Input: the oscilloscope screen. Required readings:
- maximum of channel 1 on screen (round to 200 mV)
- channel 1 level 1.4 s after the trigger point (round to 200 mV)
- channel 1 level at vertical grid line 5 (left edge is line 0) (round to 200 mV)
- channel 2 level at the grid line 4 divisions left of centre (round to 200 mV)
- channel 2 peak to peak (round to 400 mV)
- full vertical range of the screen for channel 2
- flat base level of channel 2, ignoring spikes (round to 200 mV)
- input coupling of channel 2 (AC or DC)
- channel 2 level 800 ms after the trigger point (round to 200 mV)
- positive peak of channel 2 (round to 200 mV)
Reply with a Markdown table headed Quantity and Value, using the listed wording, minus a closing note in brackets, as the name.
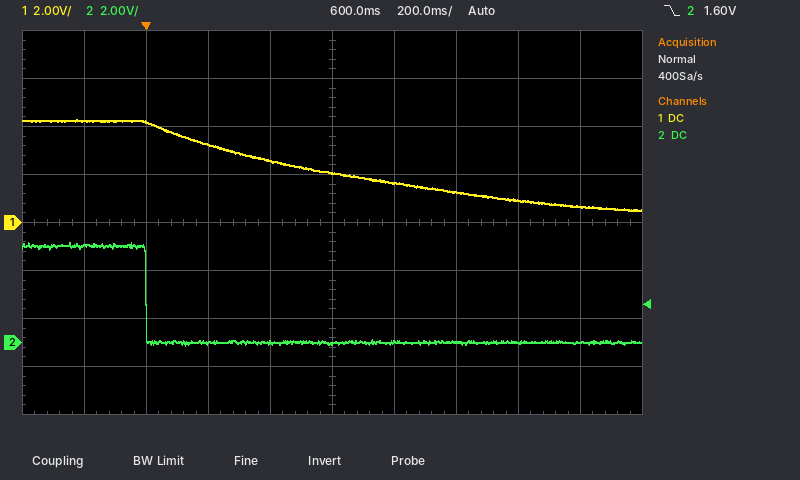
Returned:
| Quantity | Value |
|---|---|
| maximum of channel 1 on screen | 4.2 V |
| channel 1 level 1.4 s after the trigger point | 600 mV |
| channel 1 level at vertical grid line 5 (left edge is line 0) | 2.0 V |
| channel 2 level at the grid line 4 divisions left of centre | 4.0 V |
| channel 2 peak to peak | 4.4 V |
| full vertical range of the screen for channel 2 | 16 V |
| flat base level of channel 2, ignoring spikes | 0.0 V |
| input coupling of channel 2 | DC |
| channel 2 level 800 ms after the trigger point | 0.0 V |
| positive peak of channel 2 | 4.2 V |
